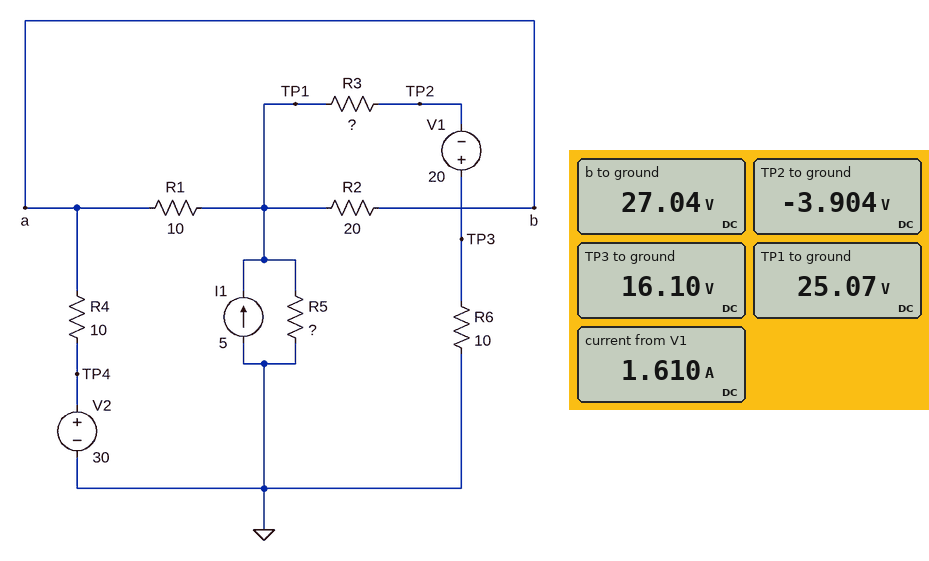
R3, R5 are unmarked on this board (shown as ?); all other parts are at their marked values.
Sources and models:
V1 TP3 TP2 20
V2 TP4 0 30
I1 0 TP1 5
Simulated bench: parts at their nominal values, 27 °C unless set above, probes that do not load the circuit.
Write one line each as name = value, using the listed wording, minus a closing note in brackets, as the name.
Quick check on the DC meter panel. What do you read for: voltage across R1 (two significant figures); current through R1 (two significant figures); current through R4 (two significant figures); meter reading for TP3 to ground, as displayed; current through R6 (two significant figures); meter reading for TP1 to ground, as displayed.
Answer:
voltage across R1 = 2.0 V
current through R1 = 200 mA
current through R4 = 300 mA
meter reading for TP3 to ground, as displayed = 16.10 V
current through R6 = 1.6 A
meter reading for TP1 to ground, as displayed = 25.07 V
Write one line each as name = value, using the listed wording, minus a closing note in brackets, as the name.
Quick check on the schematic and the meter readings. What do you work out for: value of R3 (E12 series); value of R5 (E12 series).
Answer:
value of R3 = 18 Ω
value of R5 = 6.8 Ω
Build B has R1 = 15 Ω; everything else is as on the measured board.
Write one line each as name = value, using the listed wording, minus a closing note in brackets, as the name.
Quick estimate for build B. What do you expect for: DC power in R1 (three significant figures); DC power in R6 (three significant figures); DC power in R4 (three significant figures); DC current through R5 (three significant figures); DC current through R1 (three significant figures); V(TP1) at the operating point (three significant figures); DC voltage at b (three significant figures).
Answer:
DC power in R1 = 364 mW
DC power in R6 = 25.8 W
DC power in R4 = 743 mW
DC current through R5 = 3.67 A
DC current through R1 = 156 mA
V(TP1) at the operating point = 24.9 V
DC voltage at b = 27.3 V
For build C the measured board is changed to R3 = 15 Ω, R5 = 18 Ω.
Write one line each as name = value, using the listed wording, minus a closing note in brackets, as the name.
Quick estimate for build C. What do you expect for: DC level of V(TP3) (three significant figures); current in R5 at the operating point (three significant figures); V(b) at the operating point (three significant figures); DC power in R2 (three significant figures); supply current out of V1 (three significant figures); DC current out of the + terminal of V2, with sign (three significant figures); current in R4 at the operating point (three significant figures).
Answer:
DC level of V(TP3) = 23.4 V
current in R5 at the operating point = 2.14 A
V(b) at the operating point = 35.1 V
DC power in R2 = 588 mW
supply current out of V1 = 2.34 A
DC current out of the + terminal of V2, with sign = -514 mA
current in R4 at the operating point = 514 mA
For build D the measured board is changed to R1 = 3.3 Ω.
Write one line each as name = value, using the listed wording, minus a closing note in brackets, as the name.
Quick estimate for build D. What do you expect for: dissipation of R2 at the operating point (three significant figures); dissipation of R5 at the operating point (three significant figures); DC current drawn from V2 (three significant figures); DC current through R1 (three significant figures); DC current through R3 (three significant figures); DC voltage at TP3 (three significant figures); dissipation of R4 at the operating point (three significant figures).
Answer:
dissipation of R2 at the operating point = 51.4 mW
dissipation of R5 at the operating point = 94.9 W
DC current drawn from V2 = 358 mA
DC current through R1 = 307 mA
DC current through R3 = 1.62 A
DC voltage at TP3 = 16.2 V
dissipation of R4 at the operating point = 1.28 W
